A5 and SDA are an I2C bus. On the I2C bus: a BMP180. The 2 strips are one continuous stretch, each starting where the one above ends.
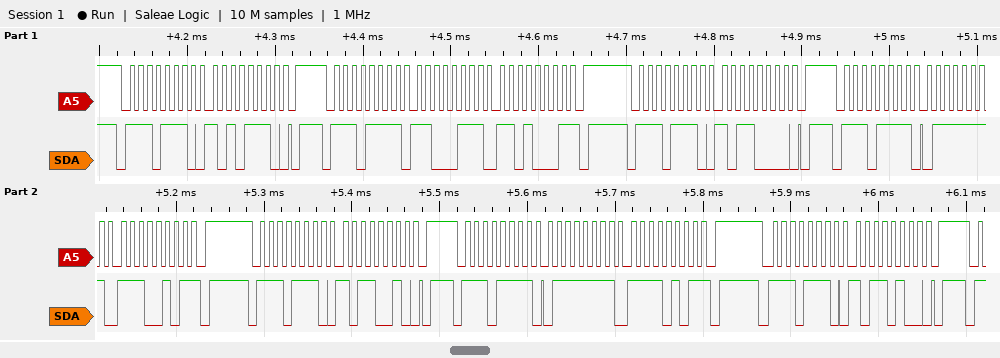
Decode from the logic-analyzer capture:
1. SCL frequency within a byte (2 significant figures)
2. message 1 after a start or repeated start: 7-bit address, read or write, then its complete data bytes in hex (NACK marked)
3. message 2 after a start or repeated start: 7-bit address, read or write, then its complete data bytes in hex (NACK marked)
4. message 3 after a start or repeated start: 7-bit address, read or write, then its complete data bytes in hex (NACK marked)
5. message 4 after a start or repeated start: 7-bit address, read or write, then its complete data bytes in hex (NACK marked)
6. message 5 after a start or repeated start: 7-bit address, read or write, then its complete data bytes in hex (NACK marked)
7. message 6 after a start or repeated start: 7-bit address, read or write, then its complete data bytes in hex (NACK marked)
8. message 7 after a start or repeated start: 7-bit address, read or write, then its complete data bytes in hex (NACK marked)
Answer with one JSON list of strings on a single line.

["100 kHz", "0x77 write: AE", "0x77 read: C7 D1 NACK", "0x77 write: B0", "0x77 read: 7F E5 NACK", "0x77 write: B2", "0x77 read: 7F F5 NACK", "0x77 write: B4"]
